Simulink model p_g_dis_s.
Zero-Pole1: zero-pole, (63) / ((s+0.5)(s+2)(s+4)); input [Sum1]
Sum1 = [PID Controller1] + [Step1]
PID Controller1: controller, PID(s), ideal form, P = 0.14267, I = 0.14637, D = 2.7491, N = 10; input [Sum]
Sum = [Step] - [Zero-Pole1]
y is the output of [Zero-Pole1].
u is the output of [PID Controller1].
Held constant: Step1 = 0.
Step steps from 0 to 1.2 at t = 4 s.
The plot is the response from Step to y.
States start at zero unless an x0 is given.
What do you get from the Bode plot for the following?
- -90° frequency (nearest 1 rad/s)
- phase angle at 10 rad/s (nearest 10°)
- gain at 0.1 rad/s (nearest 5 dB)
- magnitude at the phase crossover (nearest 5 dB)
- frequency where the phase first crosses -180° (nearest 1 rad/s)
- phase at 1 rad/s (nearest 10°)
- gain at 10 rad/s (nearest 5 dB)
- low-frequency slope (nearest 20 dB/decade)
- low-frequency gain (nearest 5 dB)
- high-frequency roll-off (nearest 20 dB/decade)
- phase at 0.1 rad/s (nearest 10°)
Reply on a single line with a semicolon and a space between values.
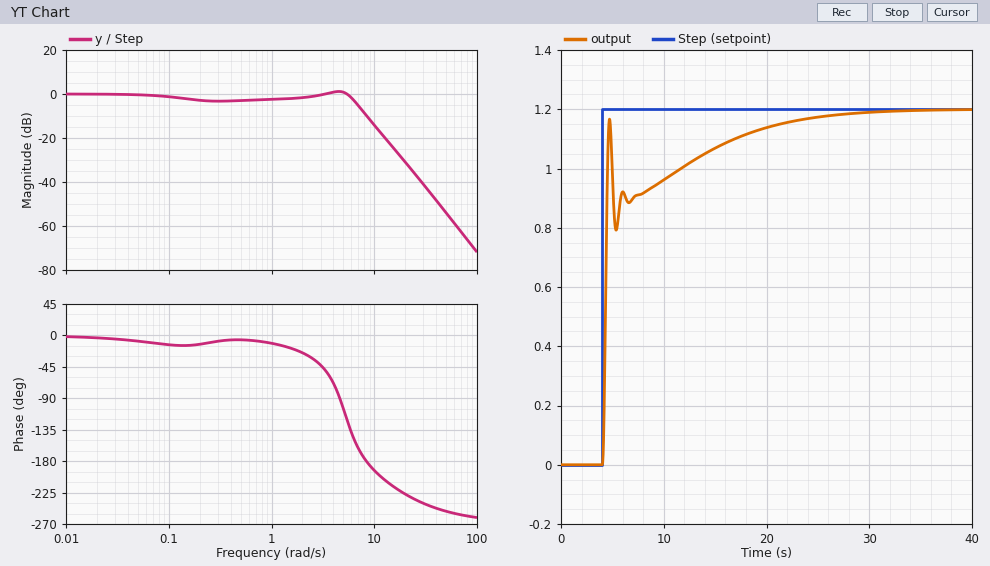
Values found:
5 rad/s; -190°; 0 dB; -10 dB; 8 rad/s; -10°; -15 dB; 0 dB/decade; 0 dB; -60 dB/decade; -10°
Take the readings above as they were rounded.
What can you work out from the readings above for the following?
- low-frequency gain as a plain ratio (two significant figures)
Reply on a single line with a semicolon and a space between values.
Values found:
1.0
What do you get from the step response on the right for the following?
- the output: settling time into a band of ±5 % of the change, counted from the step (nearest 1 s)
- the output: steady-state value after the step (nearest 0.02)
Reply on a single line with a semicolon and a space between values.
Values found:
16 s; 1.20
